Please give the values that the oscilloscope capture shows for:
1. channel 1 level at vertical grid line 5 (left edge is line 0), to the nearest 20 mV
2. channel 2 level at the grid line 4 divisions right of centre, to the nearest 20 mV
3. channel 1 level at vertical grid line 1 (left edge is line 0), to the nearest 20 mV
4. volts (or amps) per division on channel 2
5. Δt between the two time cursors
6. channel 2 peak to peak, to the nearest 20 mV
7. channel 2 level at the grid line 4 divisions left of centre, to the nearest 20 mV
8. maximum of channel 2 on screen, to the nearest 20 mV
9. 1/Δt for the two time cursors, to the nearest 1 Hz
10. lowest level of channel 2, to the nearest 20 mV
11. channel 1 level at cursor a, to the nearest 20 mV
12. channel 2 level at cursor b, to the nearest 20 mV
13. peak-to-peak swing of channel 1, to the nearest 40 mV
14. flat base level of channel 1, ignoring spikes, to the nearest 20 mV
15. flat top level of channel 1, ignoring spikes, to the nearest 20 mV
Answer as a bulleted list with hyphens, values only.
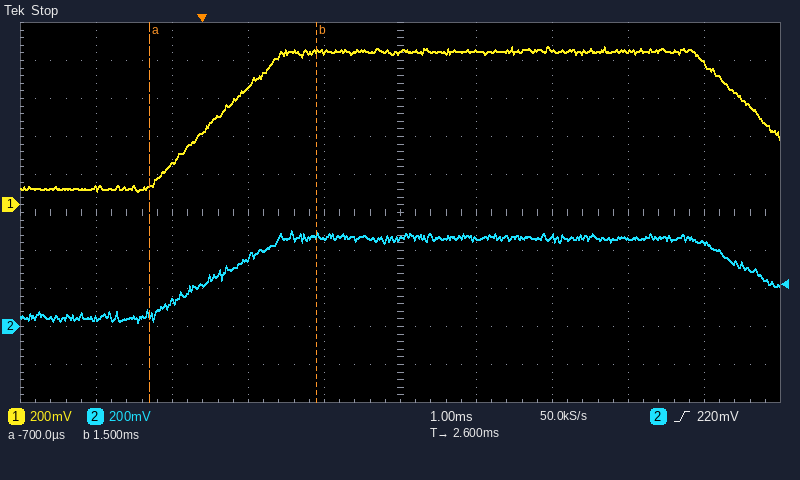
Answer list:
- 800 mV
- 440 mV
- 80 mV
- 200 mV
- 2.2 ms
- 480 mV
- 40 mV
- 500 mV
- 455 Hz
- 20 mV
- 100 mV
- 480 mV
- 760 mV
- 80 mV
- 800 mV
